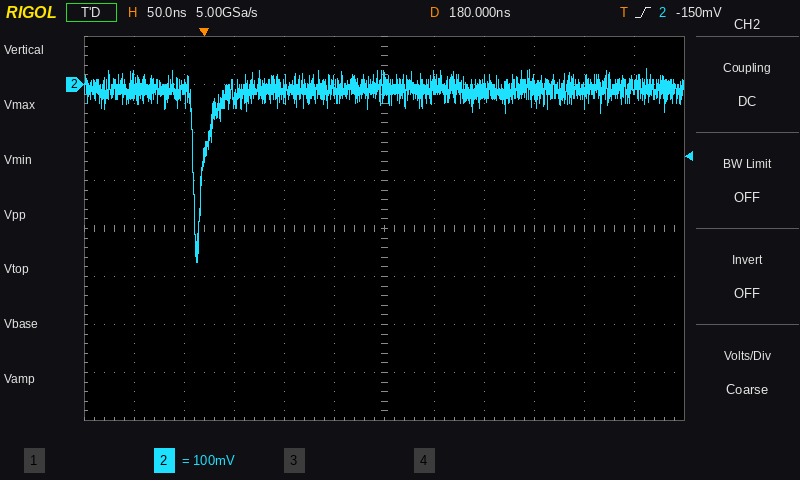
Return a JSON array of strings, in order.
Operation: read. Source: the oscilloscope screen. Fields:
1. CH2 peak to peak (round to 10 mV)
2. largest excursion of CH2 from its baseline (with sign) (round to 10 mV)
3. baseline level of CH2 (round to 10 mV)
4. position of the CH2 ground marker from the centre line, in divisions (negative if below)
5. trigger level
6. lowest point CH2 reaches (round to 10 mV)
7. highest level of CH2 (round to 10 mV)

["400 mV", "-360 mV", "-10 mV", "+3.0 div", "-150 mV", "-370 mV", "30 mV"]
